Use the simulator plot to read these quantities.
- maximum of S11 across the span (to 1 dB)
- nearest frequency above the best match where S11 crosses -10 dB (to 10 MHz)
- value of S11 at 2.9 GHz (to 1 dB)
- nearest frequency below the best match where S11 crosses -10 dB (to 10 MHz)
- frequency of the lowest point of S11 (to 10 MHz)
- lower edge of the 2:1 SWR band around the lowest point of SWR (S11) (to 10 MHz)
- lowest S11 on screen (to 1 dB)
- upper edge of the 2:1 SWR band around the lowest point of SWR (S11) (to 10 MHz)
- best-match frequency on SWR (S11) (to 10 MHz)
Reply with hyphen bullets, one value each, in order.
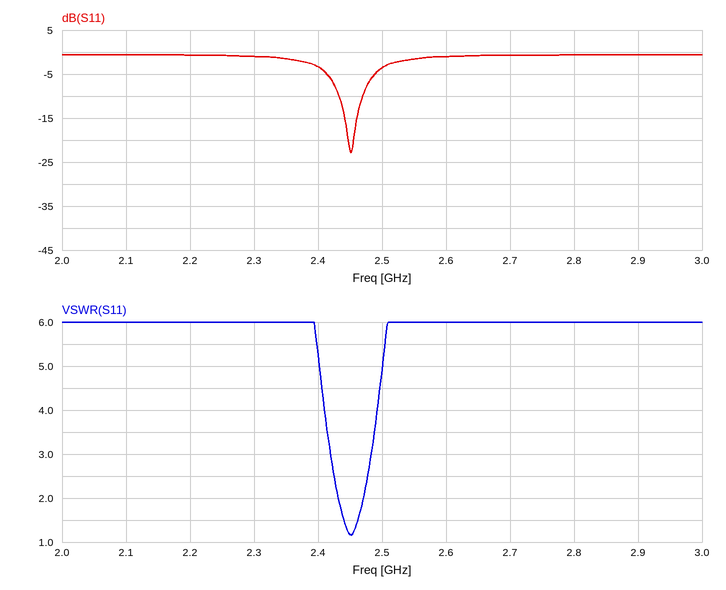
- -1 dB
- 2.47 GHz
- -1 dB
- 2.43 GHz
- 2.45 GHz
- 2.43 GHz
- -23 dB
- 2.47 GHz
- 2.45 GHz
